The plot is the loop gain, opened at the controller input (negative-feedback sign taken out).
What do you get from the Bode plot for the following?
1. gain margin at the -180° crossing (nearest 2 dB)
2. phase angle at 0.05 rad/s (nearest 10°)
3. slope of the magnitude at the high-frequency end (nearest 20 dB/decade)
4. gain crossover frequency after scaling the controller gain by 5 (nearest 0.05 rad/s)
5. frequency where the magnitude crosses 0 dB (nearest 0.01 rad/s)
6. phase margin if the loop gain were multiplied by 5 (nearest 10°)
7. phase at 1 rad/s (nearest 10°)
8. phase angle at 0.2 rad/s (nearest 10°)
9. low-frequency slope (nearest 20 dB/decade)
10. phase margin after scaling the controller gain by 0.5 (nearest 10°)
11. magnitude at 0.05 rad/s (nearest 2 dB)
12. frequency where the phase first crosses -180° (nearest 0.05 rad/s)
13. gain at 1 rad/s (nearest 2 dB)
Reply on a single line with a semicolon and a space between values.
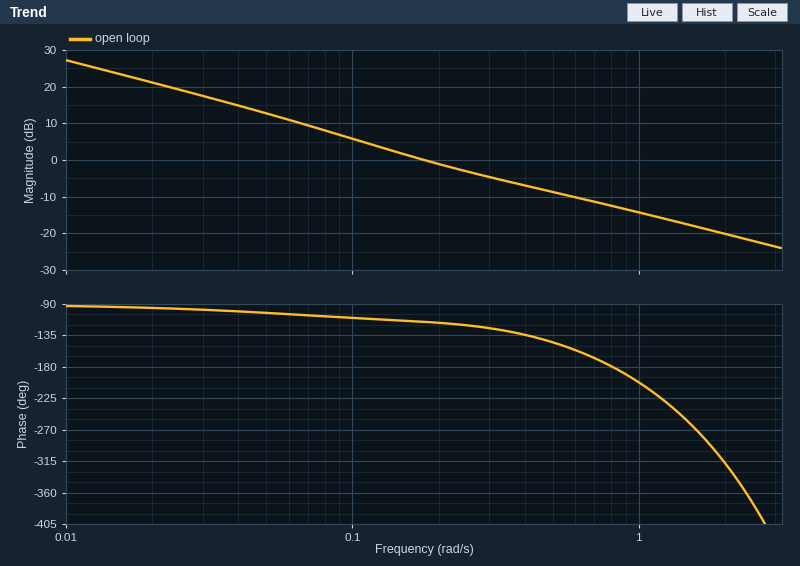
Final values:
12 dB; -100°; -20 dB/decade; 0.95 rad/s; 0.18 rad/s; -20°; -200°; -120°; -20 dB/decade; 70°; 12 dB; 0.80 rad/s; -14 dB
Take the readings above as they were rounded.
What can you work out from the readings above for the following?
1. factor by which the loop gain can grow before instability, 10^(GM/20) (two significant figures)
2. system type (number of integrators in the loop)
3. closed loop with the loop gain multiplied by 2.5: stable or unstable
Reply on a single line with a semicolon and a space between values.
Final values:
4.0; 1; stable
